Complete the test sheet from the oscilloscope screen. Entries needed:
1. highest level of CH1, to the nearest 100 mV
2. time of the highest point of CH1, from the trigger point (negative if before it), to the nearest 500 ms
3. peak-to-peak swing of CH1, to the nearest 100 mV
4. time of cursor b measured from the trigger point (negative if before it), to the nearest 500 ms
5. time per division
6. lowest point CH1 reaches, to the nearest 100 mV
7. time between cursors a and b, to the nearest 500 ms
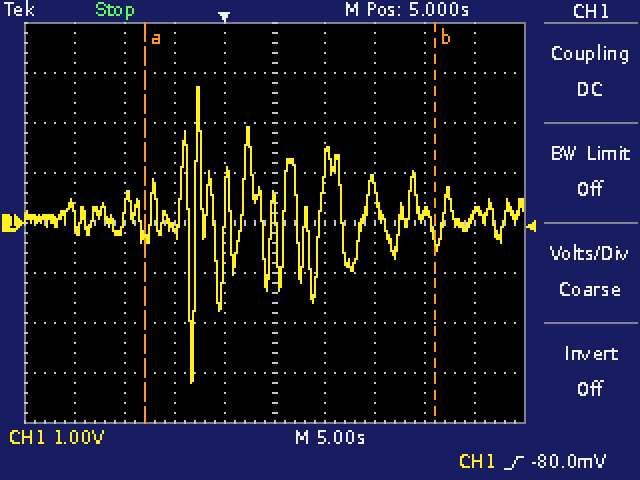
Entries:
2.7 V
-2.5 s
5.9 V
+21.0 s
5 s
-3.2 V
29.0 s
